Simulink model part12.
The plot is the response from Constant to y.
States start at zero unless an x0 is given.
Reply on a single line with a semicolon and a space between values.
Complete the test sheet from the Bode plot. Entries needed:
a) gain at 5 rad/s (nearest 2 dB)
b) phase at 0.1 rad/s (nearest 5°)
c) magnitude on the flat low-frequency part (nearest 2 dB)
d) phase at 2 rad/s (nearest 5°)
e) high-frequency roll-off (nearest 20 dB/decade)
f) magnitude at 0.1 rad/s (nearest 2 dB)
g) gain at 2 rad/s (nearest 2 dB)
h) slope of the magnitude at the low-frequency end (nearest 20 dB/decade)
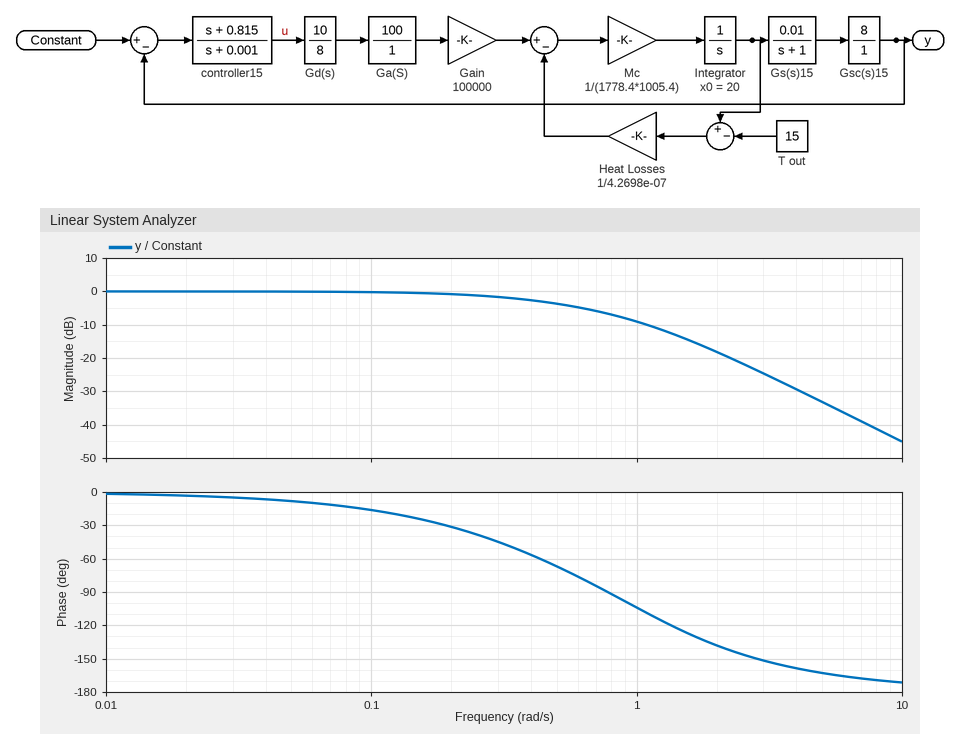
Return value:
-34 dB; -15°; 0 dB; -140°; -40 dB/decade; 0 dB; -18 dB; 0 dB/decade
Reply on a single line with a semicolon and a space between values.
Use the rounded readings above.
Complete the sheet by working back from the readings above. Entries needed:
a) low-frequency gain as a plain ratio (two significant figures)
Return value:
1.0
